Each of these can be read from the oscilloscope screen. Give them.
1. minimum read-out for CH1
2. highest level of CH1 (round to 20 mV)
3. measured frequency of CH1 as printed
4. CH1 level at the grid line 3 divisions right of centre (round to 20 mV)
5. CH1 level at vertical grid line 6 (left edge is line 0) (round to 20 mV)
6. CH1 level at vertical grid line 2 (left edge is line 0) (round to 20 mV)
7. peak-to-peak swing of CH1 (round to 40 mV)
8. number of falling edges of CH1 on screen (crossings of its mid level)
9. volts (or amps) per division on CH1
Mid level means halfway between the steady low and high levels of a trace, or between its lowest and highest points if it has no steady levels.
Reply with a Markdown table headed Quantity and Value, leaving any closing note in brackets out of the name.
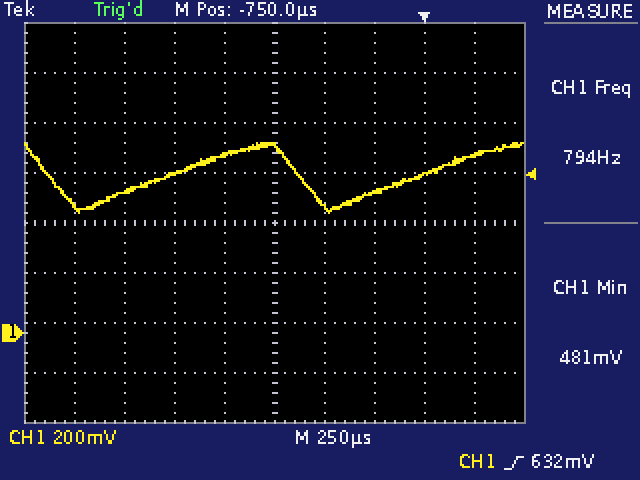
| Quantity | Value |
|---|---|
| minimum read-out for CH1 | 481 mV |
| highest level of CH1 | 760 mV |
| measured frequency of CH1 as printed | 794 Hz |
| CH1 level at the grid line 3 divisions right of centre | 640 mV |
| CH1 level at vertical grid line 6 (left edge is line 0) | 500 mV |
| CH1 level at vertical grid line 2 (left edge is line 0) | 560 mV |
| peak-to-peak swing of CH1 | 280 mV |
| number of falling edges of CH1 on screen | 2 |
| volts (or amps) per division on CH1 | 200 mV |
